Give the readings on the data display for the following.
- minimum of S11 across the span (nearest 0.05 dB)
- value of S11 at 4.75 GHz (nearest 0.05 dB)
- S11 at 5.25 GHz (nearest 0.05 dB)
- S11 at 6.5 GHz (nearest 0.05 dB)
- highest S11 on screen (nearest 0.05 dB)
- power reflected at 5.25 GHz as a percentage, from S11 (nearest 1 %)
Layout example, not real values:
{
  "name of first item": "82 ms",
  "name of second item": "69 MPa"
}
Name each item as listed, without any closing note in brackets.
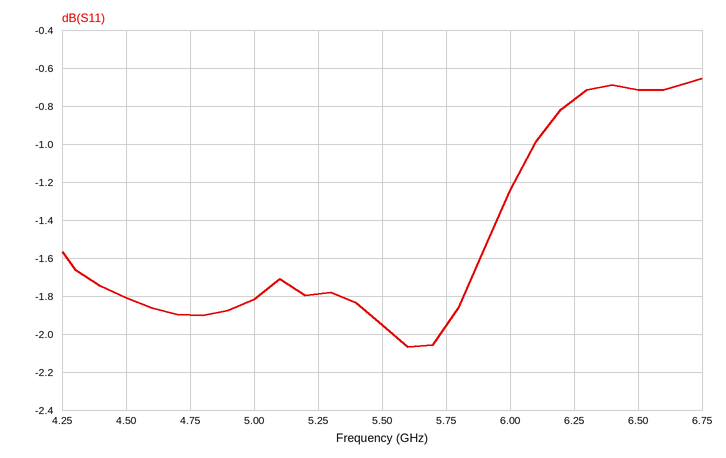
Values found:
{
  "minimum of S11 across the span": "-2.05 dB",
  "value of S11 at 4.75 GHz": "-1.90 dB",
  "S11 at 5.25 GHz": "-1.80 dB",
  "S11 at 6.5 GHz": "-0.70 dB",
  "highest S11 on screen": "-0.65 dB",
  "power reflected at 5.25 GHz as a percentage, from S11": "66 %"
}
